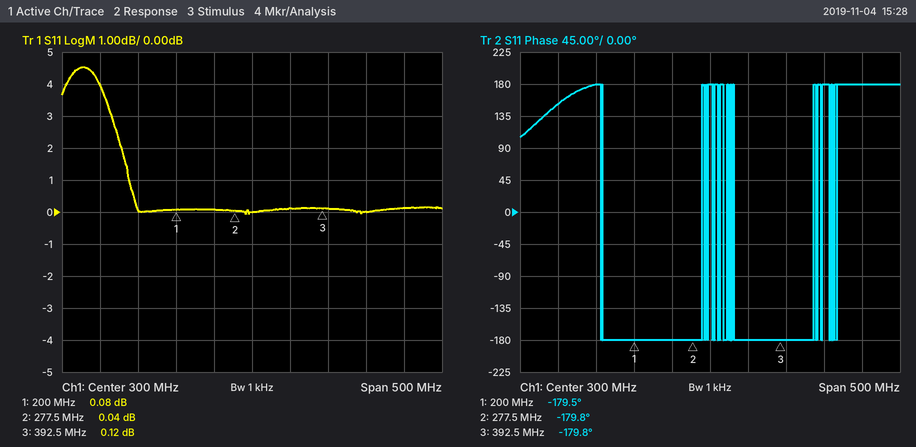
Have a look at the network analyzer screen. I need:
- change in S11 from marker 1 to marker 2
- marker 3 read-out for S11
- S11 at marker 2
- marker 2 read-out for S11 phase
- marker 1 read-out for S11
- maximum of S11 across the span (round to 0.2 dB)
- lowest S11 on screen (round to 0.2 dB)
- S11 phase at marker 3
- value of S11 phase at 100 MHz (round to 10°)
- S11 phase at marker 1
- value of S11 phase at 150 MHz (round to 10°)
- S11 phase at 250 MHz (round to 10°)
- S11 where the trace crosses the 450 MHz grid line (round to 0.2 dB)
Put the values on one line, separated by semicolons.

-0.04 dB; 0.12 dB; 0.04 dB; -179.8°; 0.08 dB; 4.6 dB; 0.0 dB; -179.8°; 150°; -179.5°; 180°; -180°; 0.0 dB
